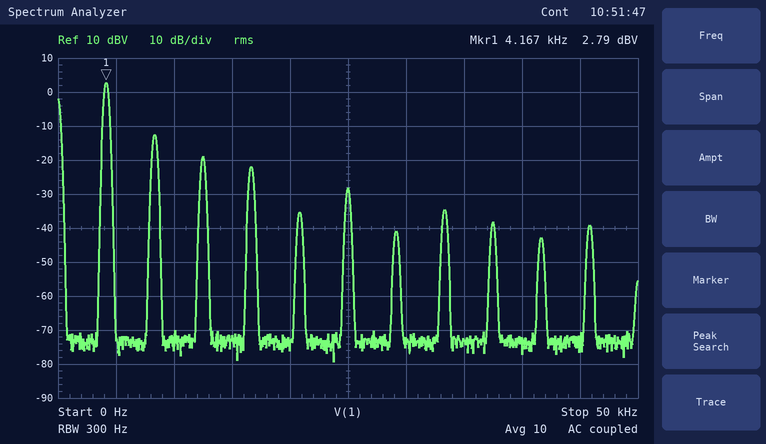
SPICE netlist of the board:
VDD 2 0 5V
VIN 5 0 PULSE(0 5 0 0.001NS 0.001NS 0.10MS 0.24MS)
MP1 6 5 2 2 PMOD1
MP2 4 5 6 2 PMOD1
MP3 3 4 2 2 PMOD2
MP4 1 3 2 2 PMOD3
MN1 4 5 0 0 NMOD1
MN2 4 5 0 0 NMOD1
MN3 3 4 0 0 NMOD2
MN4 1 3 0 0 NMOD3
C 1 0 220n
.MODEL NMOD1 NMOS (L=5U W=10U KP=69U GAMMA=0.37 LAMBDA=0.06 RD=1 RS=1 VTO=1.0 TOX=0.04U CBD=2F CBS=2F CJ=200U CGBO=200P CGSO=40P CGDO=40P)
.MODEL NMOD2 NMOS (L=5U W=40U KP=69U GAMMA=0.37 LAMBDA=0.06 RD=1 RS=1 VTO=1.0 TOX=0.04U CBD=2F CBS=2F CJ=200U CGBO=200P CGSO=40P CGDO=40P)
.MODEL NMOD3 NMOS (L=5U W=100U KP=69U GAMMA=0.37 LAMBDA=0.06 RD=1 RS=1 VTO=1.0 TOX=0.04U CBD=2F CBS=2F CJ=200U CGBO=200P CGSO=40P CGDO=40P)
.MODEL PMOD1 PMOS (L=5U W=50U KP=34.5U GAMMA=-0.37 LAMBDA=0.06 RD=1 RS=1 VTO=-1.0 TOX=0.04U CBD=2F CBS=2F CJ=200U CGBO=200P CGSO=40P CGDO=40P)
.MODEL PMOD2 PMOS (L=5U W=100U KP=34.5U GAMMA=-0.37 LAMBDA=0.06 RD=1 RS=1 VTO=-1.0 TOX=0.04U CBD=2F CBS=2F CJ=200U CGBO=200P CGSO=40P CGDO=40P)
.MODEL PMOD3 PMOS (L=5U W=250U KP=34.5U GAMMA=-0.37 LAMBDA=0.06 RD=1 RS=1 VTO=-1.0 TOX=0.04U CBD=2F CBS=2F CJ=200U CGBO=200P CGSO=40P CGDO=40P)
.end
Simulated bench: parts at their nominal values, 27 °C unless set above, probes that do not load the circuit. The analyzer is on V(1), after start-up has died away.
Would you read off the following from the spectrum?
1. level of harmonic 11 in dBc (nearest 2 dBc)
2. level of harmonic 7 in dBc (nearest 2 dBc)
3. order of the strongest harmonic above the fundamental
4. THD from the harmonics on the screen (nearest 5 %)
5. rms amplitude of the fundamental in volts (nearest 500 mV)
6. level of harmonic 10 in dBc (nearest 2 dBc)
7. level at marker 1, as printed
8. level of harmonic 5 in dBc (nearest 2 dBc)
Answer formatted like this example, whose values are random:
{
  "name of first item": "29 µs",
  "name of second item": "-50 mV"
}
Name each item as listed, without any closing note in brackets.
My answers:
{
  "level of harmonic 11 in dBc": "-42 dBc",
  "level of harmonic 7 in dBc": "-44 dBc",
  "order of the strongest harmonic above the fundamental": "2",
  "THD from the harmonics on the screen": "20 %",
  "rms amplitude of the fundamental in volts": "1.5 V",
  "level of harmonic 10 in dBc": "-46 dBc",
  "level at marker 1, as printed": "2.79 dBV",
  "level of harmonic 5 in dBc": "-38 dBc"
}
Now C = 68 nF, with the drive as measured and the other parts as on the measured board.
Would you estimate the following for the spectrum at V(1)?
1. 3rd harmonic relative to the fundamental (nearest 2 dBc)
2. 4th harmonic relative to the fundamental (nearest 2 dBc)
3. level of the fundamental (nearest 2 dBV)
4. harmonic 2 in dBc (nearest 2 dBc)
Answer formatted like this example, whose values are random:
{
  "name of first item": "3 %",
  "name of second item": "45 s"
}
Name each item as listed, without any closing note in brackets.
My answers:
{
  "3rd harmonic relative to the fundamental": "-16 dBc",
  "4th harmonic relative to the fundamental": "-18 dBc",
  "level of the fundamental": "6 dBV",
  "harmonic 2 in dBc": "-12 dBc"
}
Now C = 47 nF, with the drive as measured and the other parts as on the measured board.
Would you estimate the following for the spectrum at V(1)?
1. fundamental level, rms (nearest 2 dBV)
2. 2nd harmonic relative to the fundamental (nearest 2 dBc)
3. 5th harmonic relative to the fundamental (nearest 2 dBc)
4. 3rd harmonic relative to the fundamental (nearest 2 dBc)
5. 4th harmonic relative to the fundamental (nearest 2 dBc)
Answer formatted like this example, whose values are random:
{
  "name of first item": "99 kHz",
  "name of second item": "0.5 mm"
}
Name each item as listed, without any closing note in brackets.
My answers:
{
  "fundamental level, rms": "6 dBV",
  "2nd harmonic relative to the fundamental": "-12 dBc",
  "5th harmonic relative to the fundamental": "-32 dBc",
  "3rd harmonic relative to the fundamental": "-14 dBc",
  "4th harmonic relative to the fundamental": "-16 dBc"
}
